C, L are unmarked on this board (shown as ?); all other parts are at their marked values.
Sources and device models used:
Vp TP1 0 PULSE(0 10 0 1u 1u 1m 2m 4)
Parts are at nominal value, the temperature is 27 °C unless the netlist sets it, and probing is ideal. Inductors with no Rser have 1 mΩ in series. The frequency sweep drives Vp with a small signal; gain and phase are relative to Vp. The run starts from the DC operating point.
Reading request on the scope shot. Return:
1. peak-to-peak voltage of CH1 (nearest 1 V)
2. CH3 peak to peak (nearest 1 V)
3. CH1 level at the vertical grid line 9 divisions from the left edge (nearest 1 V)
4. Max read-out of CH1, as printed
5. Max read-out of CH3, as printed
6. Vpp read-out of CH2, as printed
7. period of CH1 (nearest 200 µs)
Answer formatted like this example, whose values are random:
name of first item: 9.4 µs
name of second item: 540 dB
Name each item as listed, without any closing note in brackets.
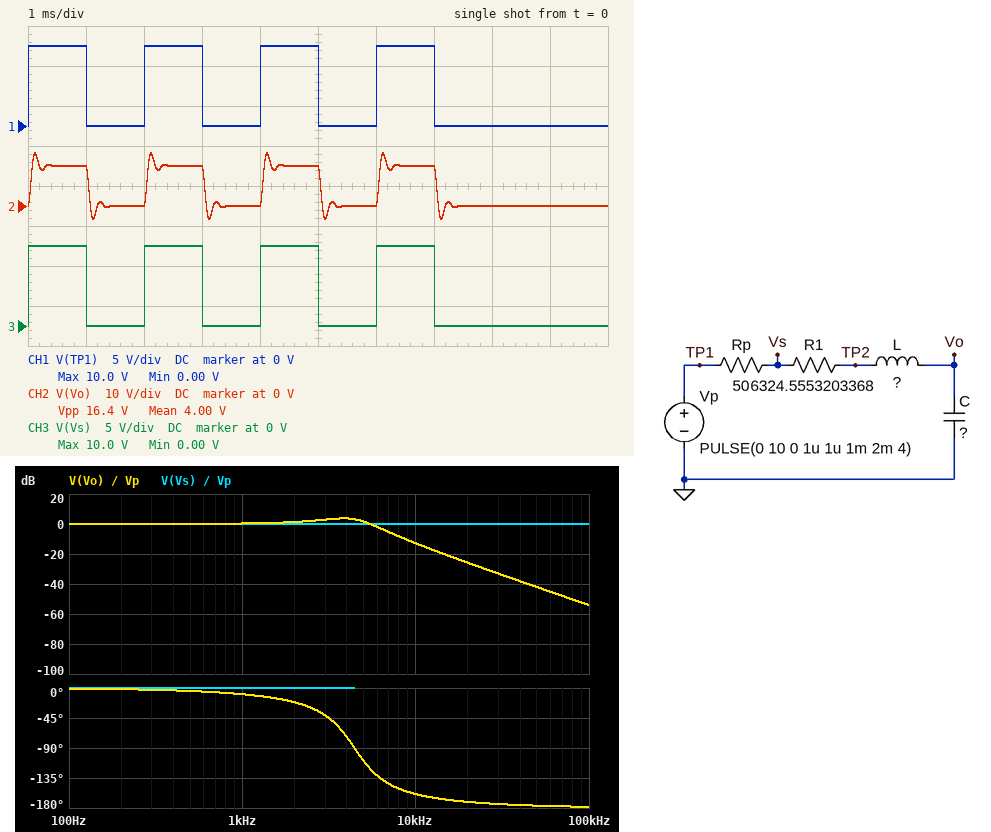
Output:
peak-to-peak voltage of CH1: 10 V
CH3 peak to peak: 10 V
CH1 level at the vertical grid line 9 divisions from the left edge: 0 V
Max read-out of CH1, as printed: 10.0 V
Max read-out of CH3, as printed: 10.0 V
Vpp read-out of CH2, as printed: 16.4 V
period of CH1: 2.0 ms
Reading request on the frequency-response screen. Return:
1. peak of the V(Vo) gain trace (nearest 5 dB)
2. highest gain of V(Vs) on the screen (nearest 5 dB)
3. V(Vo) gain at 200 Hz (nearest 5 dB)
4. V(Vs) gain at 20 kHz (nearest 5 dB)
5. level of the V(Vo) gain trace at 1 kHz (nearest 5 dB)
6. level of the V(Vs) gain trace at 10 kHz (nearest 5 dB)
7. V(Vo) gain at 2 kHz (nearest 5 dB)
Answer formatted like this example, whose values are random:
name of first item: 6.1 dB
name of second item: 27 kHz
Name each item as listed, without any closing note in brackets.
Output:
peak of the V(Vo) gain trace: 5 dB
highest gain of V(Vs) on the screen: 0 dB
V(Vo) gain at 200 Hz: 0 dB
V(Vs) gain at 20 kHz: 0 dB
level of the V(Vo) gain trace at 1 kHz: 0 dB
level of the V(Vs) gain trace at 10 kHz: 0 dB
V(Vo) gain at 2 kHz: 0 dB
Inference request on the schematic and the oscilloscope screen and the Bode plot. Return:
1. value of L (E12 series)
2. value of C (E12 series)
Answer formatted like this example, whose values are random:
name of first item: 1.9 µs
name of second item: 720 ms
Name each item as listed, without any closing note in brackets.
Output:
value of L: 330 mH
value of C: 3.9 nF
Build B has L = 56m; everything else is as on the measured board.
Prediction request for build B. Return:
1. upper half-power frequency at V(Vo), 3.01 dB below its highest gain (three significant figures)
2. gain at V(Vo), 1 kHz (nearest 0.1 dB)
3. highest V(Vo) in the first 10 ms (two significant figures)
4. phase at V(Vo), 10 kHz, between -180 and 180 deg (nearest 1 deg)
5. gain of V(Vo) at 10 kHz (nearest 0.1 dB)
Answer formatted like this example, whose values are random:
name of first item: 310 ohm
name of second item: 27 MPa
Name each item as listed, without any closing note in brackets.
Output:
upper half-power frequency at V(Vo), 3.01 dB below its highest gain: 8.80 kHz
gain at V(Vo), 1 kHz: 0 dB
highest V(Vo) in the first 10 ms: 10 V
phase at V(Vo), 10 kHz, between -180 and 180 deg: -85 deg
gain of V(Vo) at 10 kHz: -3.9 dB
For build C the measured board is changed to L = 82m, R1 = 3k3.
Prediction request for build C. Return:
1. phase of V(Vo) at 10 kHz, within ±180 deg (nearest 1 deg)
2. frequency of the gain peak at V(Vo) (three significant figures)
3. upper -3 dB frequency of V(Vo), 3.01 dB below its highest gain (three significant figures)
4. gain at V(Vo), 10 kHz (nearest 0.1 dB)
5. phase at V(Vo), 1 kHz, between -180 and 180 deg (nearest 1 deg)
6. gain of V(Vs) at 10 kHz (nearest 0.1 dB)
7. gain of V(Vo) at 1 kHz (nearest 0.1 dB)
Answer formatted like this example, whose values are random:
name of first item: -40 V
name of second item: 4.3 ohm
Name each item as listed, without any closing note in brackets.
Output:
phase of V(Vo) at 10 kHz, within ±180 deg: -108 deg
frequency of the gain peak at V(Vo): 7.62 kHz
upper -3 dB frequency of V(Vo), 3.01 dB below its highest gain: 10.6 kHz
gain at V(Vo), 10 kHz: 1.3 dB
phase at V(Vo), 1 kHz, between -180 and 180 deg: -5 deg
gain of V(Vs) at 10 kHz: -0.1 dB
gain of V(Vo) at 1 kHz: 0.1 dB
